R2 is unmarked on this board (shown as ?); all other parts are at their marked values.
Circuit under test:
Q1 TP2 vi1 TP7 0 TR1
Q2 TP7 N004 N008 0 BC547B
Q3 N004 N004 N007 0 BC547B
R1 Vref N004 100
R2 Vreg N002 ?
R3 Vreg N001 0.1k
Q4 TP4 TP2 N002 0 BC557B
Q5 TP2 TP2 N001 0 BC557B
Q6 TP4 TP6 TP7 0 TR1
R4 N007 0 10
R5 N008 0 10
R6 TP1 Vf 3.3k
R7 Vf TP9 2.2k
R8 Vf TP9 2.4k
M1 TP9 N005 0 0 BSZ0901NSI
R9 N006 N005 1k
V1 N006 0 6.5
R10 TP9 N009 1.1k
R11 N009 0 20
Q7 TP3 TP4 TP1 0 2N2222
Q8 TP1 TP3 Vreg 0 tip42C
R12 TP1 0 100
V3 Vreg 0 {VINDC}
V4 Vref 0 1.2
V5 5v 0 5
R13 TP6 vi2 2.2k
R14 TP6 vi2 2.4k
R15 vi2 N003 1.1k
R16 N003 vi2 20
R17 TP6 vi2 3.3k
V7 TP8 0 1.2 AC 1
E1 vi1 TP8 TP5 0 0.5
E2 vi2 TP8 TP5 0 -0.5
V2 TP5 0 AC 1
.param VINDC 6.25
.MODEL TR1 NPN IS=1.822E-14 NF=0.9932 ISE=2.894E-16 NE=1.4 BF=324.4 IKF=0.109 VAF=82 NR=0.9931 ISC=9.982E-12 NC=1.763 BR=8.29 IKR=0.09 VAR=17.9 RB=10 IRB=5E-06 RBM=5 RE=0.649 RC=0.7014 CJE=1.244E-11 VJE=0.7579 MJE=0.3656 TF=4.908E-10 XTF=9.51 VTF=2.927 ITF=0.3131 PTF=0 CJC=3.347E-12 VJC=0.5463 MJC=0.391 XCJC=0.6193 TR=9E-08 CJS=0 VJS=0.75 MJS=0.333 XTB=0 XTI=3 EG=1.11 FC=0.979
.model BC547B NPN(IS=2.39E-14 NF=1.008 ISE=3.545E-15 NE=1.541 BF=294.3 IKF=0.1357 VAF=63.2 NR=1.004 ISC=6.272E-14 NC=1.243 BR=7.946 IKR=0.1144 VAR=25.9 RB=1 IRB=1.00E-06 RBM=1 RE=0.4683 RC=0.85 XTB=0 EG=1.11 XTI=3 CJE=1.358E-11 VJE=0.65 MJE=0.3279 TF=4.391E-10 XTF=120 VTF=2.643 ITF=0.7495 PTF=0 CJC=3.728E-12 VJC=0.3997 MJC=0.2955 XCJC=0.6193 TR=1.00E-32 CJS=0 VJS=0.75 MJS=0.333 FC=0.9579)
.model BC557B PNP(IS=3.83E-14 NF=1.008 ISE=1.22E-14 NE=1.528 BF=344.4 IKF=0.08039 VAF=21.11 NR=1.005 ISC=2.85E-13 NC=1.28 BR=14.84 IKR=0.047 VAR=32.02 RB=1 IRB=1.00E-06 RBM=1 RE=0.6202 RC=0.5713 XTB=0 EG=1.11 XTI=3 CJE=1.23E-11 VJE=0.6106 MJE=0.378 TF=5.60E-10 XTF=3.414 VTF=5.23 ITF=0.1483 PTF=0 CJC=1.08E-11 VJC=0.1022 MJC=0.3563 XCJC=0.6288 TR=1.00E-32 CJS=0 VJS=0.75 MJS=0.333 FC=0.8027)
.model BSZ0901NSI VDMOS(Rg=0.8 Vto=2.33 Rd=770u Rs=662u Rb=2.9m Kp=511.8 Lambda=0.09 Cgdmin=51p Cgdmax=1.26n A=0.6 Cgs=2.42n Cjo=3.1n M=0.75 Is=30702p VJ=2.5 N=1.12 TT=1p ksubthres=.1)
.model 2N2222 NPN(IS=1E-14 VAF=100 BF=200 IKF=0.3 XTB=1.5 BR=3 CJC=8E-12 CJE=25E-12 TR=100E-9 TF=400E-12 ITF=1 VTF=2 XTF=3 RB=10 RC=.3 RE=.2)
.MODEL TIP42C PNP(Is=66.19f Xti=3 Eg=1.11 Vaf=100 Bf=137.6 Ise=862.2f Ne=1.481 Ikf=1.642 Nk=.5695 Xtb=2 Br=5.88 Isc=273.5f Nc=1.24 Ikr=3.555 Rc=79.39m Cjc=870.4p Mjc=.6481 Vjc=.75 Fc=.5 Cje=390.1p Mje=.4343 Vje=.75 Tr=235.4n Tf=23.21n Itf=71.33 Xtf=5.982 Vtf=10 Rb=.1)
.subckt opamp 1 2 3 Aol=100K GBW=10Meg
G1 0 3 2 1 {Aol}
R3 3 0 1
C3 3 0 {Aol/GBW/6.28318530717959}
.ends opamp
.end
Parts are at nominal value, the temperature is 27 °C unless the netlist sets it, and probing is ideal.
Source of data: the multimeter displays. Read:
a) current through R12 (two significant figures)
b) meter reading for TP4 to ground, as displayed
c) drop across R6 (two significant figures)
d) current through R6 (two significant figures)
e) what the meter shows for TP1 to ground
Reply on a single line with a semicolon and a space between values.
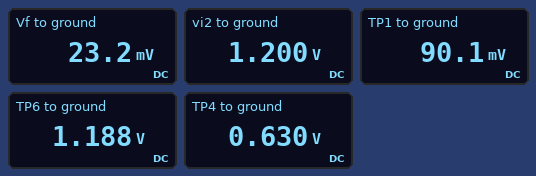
900 µA; 0.630 V; 67 mV; 20 µA; 90.1 mV
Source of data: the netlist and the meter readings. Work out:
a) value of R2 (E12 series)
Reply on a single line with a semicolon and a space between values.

180 Ω
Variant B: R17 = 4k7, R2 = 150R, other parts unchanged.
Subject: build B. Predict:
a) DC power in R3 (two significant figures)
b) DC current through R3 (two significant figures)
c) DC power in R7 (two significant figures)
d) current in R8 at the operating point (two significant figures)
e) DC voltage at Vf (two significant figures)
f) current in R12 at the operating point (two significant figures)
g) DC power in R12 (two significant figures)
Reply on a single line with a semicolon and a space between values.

750 µW; 2.7 mA; 460 nW; 13 µA; 32 mV; 1.2 mA; 150 µW
